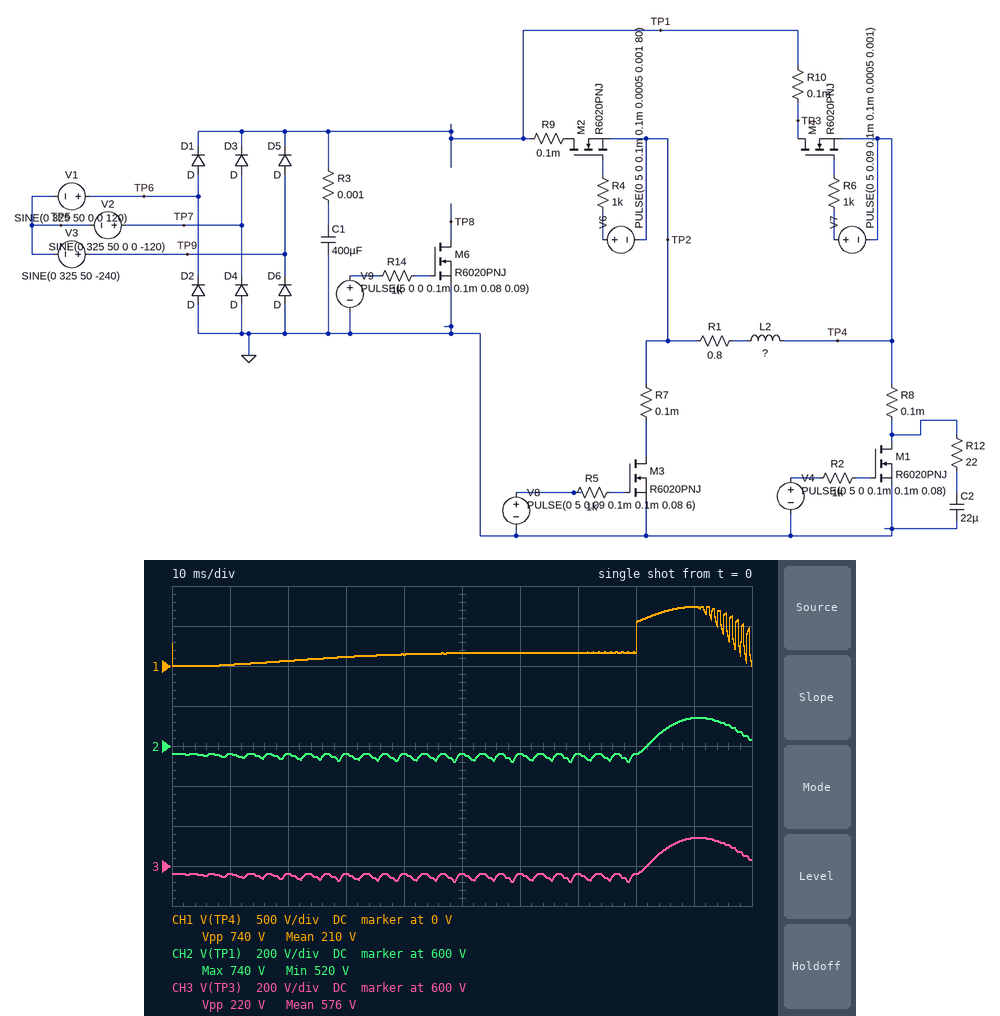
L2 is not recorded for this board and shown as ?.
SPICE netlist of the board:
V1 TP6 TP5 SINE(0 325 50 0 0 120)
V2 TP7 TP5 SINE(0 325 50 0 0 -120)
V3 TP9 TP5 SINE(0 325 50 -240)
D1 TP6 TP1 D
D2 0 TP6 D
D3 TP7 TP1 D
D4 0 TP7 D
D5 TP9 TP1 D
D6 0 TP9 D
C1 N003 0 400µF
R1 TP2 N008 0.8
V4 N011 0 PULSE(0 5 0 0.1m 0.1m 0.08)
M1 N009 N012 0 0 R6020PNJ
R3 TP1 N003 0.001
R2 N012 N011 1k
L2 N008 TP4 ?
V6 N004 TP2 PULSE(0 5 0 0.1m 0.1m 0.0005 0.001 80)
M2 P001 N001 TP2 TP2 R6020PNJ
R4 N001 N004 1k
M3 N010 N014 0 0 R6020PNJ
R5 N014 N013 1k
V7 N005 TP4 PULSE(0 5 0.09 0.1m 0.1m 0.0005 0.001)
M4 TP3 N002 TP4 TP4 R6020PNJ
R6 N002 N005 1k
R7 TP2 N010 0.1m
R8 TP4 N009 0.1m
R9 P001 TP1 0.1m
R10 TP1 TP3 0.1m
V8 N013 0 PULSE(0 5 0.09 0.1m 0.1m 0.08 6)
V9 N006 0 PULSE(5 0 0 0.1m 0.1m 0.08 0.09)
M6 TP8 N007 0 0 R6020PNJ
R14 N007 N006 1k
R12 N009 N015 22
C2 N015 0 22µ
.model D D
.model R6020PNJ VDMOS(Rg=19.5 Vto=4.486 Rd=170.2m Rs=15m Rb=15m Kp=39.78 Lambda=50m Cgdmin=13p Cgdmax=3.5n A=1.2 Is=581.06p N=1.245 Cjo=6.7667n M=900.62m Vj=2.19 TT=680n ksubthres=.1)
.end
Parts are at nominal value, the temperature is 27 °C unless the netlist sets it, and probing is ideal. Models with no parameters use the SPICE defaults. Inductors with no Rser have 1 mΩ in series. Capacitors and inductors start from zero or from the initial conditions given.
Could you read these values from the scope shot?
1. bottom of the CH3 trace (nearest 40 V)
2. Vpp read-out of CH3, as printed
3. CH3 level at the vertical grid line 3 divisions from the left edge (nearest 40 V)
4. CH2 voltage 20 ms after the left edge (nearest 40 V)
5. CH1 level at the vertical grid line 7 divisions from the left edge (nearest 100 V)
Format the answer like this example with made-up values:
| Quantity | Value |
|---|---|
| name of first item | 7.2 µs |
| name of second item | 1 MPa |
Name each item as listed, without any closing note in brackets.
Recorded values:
| Quantity | Value |
|---|---|
| bottom of the CH3 trace | 520 V |
| Vpp read-out of CH3, as printed | 220 V |
| CH3 level at the vertical grid line 3 divisions from the left edge | 560 V |
| CH2 voltage 20 ms after the left edge | 560 V |
| CH1 level at the vertical grid line 7 divisions from the left edge | 200 V |
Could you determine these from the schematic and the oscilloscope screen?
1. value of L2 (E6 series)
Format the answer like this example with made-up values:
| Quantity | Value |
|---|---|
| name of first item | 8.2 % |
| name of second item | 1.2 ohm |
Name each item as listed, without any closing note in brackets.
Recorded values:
| Quantity | Value |
|---|---|
| value of L2 | 470 mH |
